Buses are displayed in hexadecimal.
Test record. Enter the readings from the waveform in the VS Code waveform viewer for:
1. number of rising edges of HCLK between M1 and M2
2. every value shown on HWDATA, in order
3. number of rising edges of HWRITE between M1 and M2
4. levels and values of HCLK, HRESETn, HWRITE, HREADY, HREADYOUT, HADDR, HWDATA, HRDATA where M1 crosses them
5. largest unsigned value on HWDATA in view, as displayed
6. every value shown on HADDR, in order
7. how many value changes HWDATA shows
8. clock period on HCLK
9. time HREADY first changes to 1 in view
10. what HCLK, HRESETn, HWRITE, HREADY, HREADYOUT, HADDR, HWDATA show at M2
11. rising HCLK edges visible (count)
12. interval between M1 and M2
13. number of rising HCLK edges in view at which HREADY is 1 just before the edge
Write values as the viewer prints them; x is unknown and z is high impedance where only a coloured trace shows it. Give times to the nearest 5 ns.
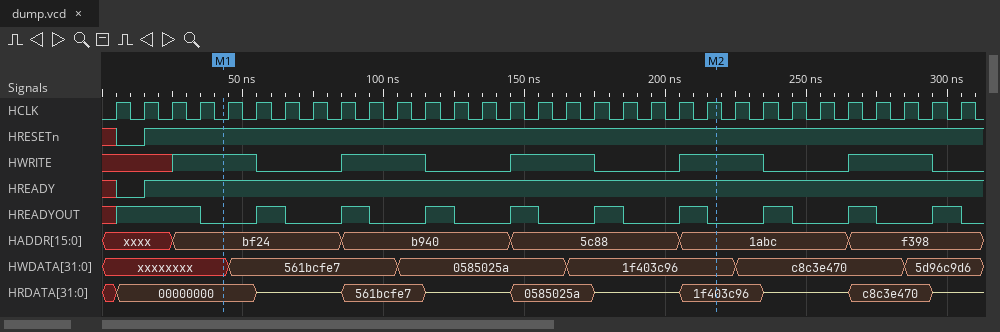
18
xxxxxxxx, 561bcfe7, 0585025a, 1f403c96, c8c3e470, 5d96c9d6
3
HCLK=0, HRESETn=1, HWRITE=1, HREADY=1, HREADYOUT=0, HADDR=bf24, HWDATA=xxxxxxxx, HRDATA=00000000
c8c3e470
xxxx, bf24, b940, 5c88, 1abc, f398
5
10 ns
15 ns
HCLK=1, HRESETn=1, HWRITE=1, HREADY=1, HREADYOUT=0, HADDR=1abc, HWDATA=1f403c96
31
175 ns
29
